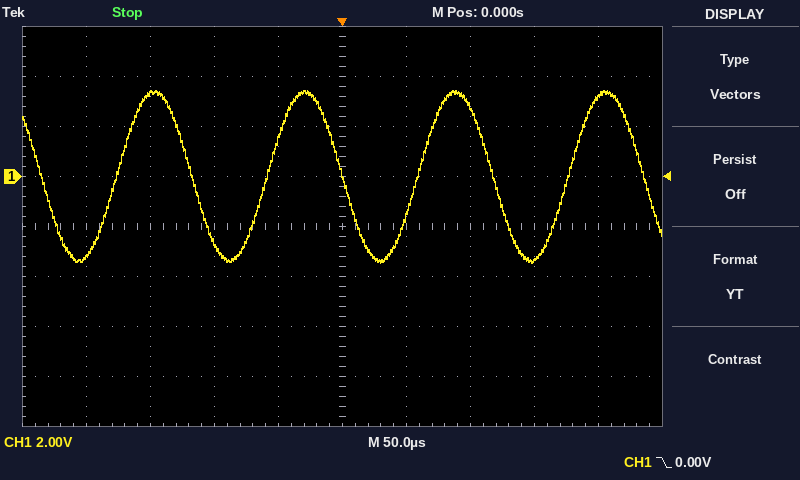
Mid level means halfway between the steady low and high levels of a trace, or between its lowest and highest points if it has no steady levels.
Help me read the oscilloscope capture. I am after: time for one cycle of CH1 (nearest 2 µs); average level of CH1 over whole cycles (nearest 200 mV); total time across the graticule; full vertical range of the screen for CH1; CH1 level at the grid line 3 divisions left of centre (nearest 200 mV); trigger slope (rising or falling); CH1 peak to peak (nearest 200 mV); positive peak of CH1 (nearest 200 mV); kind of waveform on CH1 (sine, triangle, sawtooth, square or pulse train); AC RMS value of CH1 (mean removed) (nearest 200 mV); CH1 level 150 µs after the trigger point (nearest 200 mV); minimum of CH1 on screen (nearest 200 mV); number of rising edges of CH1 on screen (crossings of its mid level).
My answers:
118 µs
0.0 V
500 µs
16 V
3.4 V
falling
6.8 V
3.4 V
sine
2.4 V
-3.4 V
-3.4 V
4
